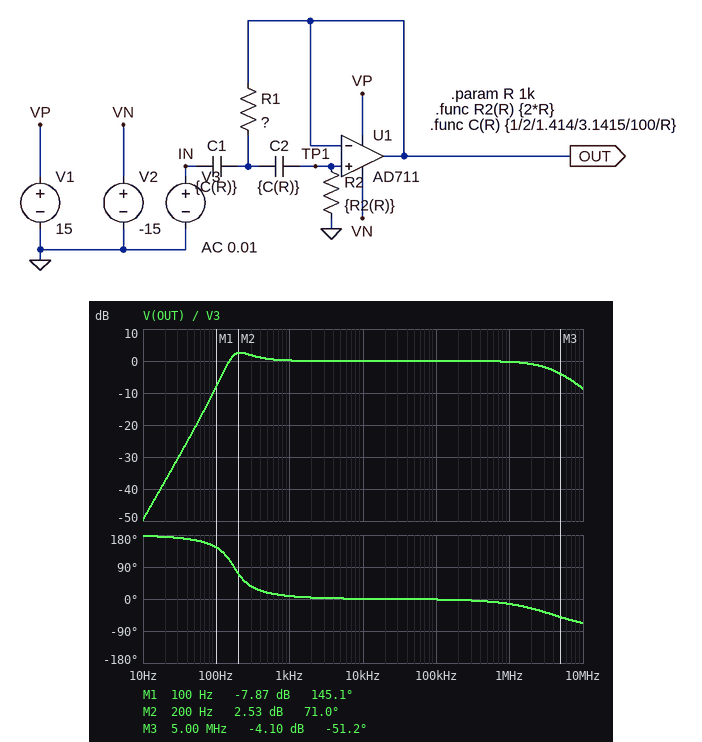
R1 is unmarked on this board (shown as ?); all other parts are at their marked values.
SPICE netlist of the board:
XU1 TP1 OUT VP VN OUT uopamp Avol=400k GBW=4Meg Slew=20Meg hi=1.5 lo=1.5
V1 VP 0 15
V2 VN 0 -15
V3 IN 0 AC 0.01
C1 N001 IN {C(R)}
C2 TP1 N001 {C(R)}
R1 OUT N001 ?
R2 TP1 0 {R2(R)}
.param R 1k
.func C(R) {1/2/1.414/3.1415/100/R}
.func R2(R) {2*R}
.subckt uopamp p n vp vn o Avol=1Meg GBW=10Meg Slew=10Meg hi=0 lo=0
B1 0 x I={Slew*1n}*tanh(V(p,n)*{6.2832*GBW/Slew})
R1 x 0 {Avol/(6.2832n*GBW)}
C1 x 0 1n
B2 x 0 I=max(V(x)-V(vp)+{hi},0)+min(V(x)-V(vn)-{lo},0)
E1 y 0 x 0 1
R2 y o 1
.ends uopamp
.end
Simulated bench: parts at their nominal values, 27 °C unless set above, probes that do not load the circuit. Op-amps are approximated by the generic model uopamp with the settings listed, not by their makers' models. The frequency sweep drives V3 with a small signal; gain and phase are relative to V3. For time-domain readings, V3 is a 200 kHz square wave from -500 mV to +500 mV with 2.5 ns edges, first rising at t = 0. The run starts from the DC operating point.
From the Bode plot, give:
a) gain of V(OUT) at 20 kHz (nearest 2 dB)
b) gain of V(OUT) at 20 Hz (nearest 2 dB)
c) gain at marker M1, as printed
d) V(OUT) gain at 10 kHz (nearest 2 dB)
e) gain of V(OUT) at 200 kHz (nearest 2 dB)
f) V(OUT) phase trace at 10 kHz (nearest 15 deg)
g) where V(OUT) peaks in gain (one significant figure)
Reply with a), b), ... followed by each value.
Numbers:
a) 0 dB
b) -38 dB
c) -7.87 dB
d) 0 dB
e) 0 dB
f) 0 deg
g) 200 Hz
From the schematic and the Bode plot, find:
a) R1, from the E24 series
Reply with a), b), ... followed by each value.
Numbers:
a) 330 Ω
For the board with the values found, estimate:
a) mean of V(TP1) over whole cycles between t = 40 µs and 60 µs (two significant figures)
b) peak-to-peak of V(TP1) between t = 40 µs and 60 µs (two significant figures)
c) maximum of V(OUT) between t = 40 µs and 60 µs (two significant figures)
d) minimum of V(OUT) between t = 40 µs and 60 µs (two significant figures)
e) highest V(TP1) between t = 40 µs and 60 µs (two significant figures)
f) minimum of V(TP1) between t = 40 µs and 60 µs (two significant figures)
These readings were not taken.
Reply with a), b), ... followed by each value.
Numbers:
a) 480 mV
b) 1.0 V
c) 980 mV
d) -27 mV
e) 980 mV
f) -27 mV
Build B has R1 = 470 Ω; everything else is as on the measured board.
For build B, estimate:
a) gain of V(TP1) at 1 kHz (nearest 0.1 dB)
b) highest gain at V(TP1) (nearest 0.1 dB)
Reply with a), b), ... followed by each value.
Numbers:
a) 0.1 dB
b) 1.4 dB
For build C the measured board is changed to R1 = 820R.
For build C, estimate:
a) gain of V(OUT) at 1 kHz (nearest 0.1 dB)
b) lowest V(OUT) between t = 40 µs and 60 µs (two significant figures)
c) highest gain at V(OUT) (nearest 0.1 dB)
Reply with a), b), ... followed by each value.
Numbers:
a) 0 dB
b) -26 mV
c) 0.1 dB
